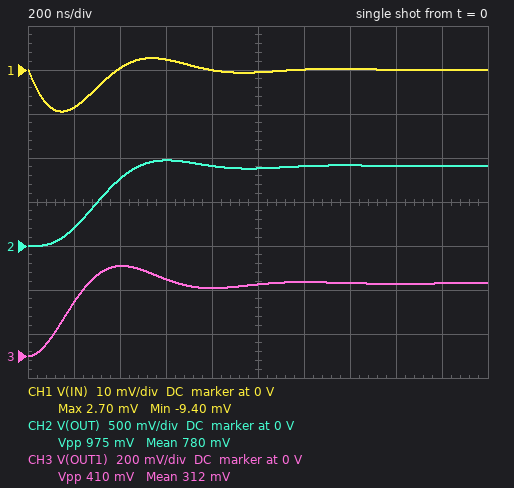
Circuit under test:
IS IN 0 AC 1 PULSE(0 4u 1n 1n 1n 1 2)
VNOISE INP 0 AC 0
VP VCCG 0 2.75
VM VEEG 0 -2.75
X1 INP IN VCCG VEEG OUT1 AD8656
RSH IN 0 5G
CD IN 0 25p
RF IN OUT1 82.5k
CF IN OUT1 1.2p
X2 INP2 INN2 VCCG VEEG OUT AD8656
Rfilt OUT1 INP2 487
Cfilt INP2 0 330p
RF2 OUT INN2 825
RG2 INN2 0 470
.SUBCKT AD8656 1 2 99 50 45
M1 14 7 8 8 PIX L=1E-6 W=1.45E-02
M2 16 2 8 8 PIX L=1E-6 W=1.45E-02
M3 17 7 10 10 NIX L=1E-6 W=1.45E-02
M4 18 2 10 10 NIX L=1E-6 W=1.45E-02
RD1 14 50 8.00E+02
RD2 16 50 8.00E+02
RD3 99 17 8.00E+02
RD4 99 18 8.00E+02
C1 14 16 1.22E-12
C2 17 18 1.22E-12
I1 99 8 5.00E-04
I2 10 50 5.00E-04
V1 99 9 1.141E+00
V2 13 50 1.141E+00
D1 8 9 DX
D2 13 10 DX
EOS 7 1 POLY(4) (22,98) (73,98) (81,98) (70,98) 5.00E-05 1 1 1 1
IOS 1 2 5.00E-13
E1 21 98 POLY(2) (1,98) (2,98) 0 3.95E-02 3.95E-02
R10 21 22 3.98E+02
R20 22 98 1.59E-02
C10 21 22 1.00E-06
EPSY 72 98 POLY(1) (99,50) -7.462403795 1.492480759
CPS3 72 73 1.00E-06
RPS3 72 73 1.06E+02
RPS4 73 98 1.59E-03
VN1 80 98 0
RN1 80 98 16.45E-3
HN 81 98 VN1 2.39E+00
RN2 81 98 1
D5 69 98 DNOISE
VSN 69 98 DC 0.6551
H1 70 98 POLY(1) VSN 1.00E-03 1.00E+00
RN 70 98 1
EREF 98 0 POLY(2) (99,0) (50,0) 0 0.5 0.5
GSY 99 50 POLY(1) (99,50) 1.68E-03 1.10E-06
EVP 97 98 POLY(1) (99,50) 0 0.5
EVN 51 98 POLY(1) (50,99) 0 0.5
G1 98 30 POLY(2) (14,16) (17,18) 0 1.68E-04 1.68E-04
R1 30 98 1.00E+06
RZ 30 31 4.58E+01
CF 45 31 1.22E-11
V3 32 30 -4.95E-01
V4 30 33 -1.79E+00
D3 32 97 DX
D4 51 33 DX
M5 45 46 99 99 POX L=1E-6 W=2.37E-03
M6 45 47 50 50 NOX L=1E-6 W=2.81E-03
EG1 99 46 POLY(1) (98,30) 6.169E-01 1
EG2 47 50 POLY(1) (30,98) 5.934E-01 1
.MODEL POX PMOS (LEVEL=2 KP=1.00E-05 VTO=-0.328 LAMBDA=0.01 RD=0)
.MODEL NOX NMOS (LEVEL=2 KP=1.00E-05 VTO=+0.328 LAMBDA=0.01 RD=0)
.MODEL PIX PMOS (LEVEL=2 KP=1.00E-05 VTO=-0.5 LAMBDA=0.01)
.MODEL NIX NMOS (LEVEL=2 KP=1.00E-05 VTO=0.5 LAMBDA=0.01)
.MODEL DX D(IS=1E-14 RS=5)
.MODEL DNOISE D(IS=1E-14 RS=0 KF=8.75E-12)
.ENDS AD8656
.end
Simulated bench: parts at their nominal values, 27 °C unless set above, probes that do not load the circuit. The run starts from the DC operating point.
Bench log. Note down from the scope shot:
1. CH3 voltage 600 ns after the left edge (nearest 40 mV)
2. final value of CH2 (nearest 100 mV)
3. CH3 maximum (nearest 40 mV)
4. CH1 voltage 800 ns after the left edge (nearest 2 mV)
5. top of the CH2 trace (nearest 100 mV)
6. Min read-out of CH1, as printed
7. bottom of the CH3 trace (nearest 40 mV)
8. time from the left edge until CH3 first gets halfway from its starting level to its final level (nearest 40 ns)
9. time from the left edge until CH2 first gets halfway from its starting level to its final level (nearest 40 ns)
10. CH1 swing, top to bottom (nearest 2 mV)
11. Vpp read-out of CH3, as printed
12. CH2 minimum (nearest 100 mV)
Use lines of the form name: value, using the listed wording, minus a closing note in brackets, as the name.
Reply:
CH3 voltage 600 ns after the left edge: 360 mV
final value of CH2: 900 mV
CH3 maximum: 400 mV
CH1 voltage 800 ns after the left edge: 0 V
top of the CH2 trace: 1.0 V
Min read-out of CH1, as printed: -9.40 mV
bottom of the CH3 trace: 0 V
time from the left edge until CH3 first gets halfway from its starting level to its final level: 160 ns
time from the left edge until CH2 first gets halfway from its starting level to its final level: 280 ns
CH1 swing, top to bottom: 12 mV
Vpp read-out of CH3, as printed: 410 mV
CH2 minimum: 0 V
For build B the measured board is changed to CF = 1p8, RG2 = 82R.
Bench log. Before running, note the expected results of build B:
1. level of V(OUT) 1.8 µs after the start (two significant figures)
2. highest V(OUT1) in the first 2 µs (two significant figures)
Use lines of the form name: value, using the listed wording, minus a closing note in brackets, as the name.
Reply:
level of V(OUT) 1.8 µs after the start: 2.7 V
highest V(OUT1) in the first 2 µs: 360 mV
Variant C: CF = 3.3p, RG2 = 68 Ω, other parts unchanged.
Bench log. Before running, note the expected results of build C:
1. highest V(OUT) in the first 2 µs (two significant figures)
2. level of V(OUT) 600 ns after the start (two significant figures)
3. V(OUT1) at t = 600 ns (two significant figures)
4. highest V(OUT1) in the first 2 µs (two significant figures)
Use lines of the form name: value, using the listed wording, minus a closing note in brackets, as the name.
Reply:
highest V(OUT) in the first 2 µs: 2.7 V
level of V(OUT) 600 ns after the start: 2.6 V
V(OUT1) at t = 600 ns: 300 mV
highest V(OUT1) in the first 2 µs: 330 mV
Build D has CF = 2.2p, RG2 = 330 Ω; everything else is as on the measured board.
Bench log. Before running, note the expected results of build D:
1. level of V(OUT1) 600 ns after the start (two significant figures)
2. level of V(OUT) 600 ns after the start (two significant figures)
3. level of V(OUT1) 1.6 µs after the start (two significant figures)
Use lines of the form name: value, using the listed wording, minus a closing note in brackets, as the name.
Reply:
level of V(OUT1) 600 ns after the start: 340 mV
level of V(OUT) 600 ns after the start: 1.0 V
level of V(OUT1) 1.6 µs after the start: 330 mV
